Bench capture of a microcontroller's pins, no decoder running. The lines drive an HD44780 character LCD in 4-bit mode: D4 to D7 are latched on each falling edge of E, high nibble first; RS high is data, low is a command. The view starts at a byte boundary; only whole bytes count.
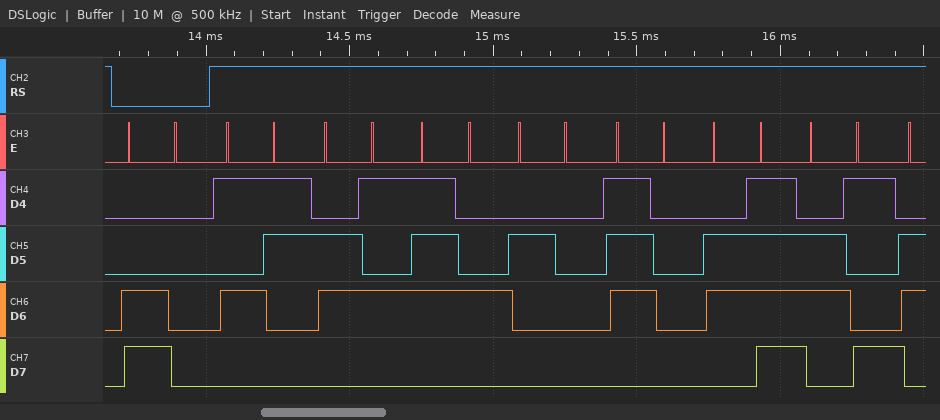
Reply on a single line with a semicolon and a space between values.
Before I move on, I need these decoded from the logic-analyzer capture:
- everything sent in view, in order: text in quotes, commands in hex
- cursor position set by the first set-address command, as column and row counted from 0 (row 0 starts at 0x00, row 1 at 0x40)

0xC0 "Set poi"; column 0, row 1
